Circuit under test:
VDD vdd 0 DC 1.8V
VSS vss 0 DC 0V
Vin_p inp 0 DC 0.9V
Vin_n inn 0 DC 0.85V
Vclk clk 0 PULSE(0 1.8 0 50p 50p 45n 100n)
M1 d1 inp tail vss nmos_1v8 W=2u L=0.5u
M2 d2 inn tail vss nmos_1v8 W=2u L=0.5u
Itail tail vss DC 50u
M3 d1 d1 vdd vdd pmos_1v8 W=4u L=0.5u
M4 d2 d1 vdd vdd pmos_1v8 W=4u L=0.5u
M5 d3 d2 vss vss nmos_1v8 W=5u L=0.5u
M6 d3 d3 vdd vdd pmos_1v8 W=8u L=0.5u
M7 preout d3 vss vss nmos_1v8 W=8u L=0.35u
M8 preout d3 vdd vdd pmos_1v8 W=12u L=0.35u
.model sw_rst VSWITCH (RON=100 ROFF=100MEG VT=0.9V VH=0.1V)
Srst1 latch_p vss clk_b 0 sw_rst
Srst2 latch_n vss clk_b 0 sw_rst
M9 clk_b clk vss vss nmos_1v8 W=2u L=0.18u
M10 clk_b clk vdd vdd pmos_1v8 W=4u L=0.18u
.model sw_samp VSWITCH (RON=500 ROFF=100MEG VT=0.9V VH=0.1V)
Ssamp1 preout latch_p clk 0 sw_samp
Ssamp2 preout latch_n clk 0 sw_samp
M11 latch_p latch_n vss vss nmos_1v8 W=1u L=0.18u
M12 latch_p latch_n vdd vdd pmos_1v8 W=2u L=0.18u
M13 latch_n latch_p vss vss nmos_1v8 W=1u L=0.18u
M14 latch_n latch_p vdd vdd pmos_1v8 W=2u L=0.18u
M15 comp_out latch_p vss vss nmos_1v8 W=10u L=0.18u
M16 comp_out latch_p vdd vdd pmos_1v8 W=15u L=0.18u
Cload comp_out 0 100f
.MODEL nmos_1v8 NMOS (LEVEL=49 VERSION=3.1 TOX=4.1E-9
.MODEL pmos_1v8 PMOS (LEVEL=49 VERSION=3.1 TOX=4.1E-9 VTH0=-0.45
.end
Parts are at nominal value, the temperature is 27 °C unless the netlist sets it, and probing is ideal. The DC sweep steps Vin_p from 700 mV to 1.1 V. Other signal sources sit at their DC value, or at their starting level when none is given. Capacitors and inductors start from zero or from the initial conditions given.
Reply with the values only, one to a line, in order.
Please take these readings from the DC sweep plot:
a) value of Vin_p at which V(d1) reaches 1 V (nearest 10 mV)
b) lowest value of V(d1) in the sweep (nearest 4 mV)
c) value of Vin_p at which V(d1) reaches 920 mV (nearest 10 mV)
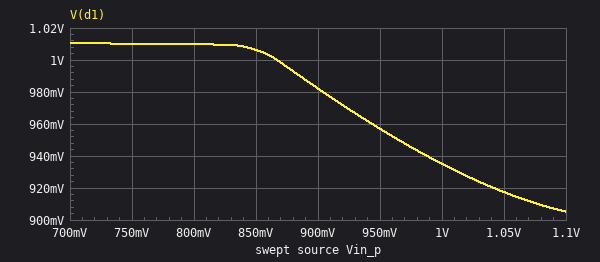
870 mV
904 mV
1.04 V
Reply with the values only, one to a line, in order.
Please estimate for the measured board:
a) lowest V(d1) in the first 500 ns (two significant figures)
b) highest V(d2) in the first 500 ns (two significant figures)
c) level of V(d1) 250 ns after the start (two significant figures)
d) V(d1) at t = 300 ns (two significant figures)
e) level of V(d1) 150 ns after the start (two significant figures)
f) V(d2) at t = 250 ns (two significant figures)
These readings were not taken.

970 mV
1.7 V
980 mV
980 mV
980 mV
1.7 V
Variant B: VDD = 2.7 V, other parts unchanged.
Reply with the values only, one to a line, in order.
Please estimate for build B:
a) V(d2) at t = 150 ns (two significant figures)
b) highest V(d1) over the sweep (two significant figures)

2.6 V
1.9 V
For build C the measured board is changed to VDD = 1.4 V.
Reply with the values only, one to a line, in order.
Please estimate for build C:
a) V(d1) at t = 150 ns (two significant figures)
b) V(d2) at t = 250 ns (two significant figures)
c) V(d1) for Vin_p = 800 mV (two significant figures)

580 mV
1.3 V
610 mV
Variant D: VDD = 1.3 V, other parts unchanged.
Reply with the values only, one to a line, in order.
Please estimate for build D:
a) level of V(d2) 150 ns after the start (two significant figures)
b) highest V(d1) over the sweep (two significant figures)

1.2 V
510 mV
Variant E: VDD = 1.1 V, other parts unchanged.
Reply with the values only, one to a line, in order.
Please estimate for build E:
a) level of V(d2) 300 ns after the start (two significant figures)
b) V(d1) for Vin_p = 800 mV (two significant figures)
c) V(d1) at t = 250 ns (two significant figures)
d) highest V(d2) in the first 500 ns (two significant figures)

780 mV
310 mV
300 mV
790 mV
